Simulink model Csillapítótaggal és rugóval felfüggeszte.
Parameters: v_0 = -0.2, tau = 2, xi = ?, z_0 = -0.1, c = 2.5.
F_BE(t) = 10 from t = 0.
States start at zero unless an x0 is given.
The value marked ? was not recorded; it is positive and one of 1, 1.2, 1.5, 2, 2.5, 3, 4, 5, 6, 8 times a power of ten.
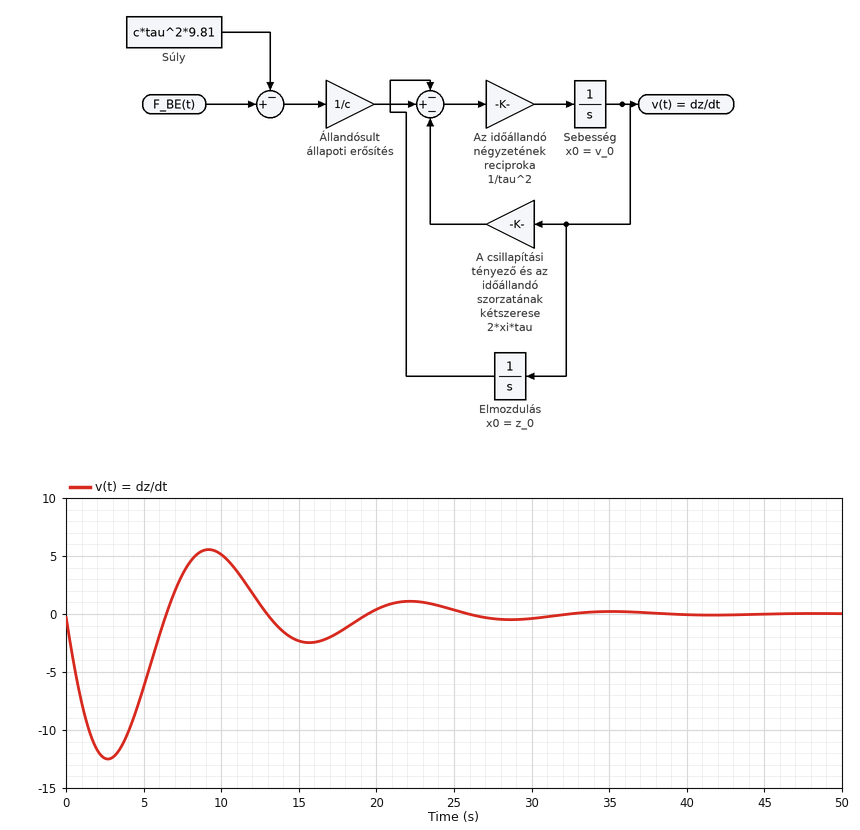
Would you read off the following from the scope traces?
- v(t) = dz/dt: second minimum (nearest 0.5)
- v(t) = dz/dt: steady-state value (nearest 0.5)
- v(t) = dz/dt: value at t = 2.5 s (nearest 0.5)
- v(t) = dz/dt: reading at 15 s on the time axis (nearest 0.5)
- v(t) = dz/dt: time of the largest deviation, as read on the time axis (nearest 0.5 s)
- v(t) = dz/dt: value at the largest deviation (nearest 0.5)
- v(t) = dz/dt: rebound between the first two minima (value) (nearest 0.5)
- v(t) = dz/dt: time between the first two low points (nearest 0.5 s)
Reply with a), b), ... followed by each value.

a) -2.5
b) 0.0
c) -12.5
d) -2.5
e) 2.5 s
f) -12.5
g) 5.5
h) 13.0 s
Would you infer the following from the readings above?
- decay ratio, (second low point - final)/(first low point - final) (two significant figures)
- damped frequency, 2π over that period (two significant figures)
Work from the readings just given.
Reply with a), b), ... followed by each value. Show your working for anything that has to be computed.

a) (-2.5 - 0) / (-12.5 - 0) = 0.20
b) 2π / 13 = 0.48 rad/s
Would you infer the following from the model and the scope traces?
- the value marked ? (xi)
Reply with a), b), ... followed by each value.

a) 0.25
